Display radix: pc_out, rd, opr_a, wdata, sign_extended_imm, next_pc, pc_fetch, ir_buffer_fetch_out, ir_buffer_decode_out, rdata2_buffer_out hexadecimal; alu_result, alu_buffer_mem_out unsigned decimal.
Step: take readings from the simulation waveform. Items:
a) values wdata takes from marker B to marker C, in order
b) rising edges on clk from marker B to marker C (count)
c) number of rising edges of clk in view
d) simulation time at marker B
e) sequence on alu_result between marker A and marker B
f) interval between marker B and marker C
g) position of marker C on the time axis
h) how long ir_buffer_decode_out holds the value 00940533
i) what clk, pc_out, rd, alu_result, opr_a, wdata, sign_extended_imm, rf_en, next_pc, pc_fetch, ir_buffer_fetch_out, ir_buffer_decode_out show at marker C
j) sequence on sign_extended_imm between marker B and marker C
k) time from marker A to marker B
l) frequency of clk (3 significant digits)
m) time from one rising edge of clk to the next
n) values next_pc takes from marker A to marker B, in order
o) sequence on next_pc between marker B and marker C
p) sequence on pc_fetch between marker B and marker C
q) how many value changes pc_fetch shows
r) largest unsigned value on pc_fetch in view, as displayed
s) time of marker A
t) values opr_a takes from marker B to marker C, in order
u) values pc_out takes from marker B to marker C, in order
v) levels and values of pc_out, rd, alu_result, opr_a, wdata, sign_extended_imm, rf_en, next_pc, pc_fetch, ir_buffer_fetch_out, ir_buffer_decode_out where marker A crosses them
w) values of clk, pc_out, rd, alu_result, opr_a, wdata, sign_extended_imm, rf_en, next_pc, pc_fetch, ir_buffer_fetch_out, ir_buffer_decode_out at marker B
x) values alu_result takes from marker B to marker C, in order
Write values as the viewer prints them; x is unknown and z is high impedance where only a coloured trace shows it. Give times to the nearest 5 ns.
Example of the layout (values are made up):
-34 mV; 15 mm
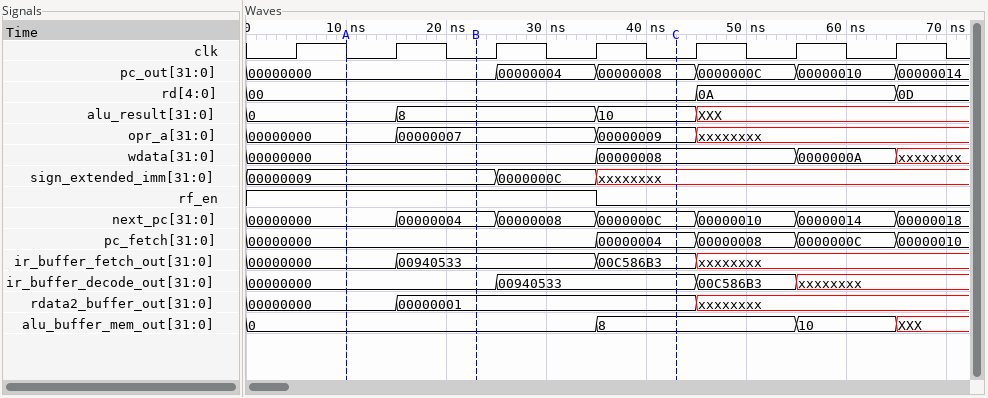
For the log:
00000000, 00000008; 2; 7; 25 ns; 0, 8; 20 ns; 45 ns; 20 ns; clk=0, pc_out=00000008, rd=00, alu_result=10, opr_a=00000009, wdata=00000008, sign_extended_imm=xxxxxxxx, rf_en=0, next_pc=0000000C, pc_fetch=00000004, ir_buffer_fetch_out=00C586B3, ir_buffer_decode_out=00940533; 00000009, 0000000C, xxxxxxxx; 15 ns; 100 MHz; 10 ns; 00000000, 00000004; 00000004, 00000008, 0000000C; 00000000, 00000004; 4; 00000010; 10 ns; 00000007, 00000009; 00000000, 00000004, 00000008; pc_out=00000000, rd=00, alu_result=0, opr_a=00000000, wdata=00000000, sign_extended_imm=00000009, rf_en=1, next_pc=00000000, pc_fetch=00000000, ir_buffer_fetch_out=00000000, ir_buffer_decode_out=00000000; clk=0, pc_out=00000000, rd=00, alu_result=8, opr_a=00000007, wdata=00000000, sign_extended_imm=00000009, rf_en=1, next_pc=00000004, pc_fetch=00000000, ir_buffer_fetch_out=00940533, ir_buffer_decode_out=00000000; 8, 10
